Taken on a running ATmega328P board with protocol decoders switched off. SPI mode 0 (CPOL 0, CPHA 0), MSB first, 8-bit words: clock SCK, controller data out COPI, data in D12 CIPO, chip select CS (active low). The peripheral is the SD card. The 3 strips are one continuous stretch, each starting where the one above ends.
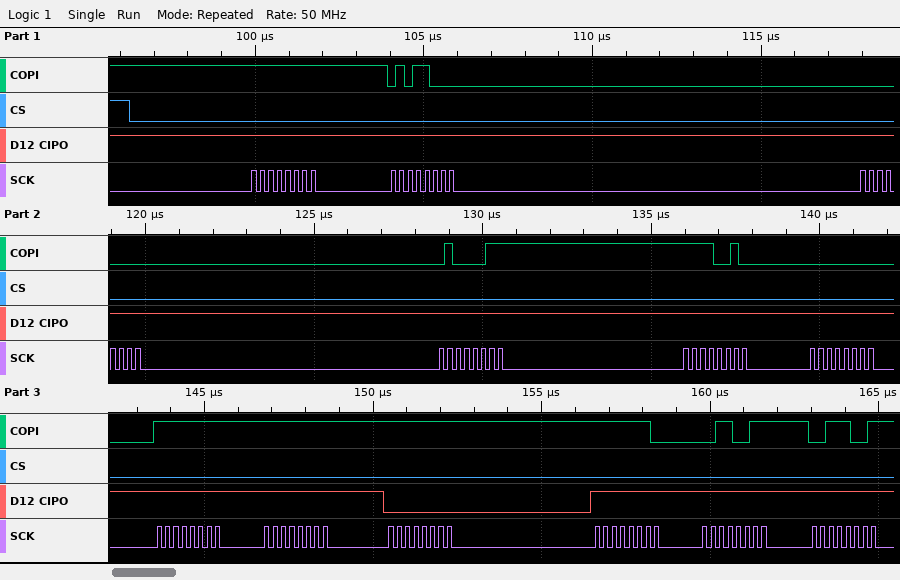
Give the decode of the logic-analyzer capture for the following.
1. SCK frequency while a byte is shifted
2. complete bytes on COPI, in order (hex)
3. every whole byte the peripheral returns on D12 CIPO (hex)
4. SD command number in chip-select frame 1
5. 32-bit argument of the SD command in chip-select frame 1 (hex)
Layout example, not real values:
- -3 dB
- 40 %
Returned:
- 4 MHz
- FF 58 00 43 F2 00 FF FF FF FE 33 39
- FF FF FF FF FF FF FF FF 00 FF FF FF
- CMD24
- 0x0043F200
